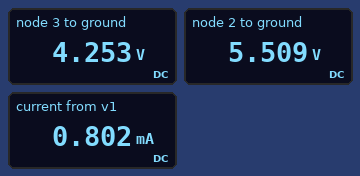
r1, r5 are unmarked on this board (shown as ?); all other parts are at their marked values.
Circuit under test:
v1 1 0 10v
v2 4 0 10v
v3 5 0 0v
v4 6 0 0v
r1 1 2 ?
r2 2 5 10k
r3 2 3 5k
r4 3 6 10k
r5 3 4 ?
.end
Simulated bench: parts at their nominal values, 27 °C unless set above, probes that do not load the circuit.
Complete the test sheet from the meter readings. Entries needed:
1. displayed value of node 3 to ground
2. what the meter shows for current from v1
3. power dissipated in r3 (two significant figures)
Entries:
4.253 V
0.802 mA
320 µW
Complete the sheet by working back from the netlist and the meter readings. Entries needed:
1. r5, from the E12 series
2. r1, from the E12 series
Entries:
33 kΩ
5.6 kΩ
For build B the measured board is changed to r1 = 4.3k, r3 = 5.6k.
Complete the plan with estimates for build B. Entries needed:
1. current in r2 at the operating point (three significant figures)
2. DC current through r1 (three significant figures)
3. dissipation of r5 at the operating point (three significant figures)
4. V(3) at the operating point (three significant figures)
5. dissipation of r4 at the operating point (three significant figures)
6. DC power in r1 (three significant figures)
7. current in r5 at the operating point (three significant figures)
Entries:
613 µA
900 µA
908 µW
4.53 V
2.05 mW
3.48 mW
166 µA
